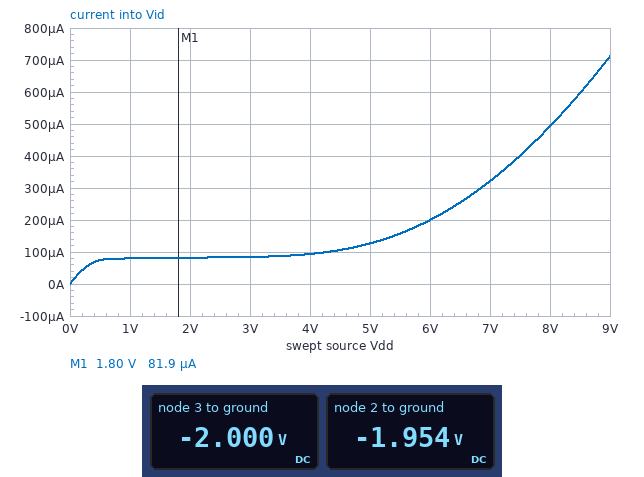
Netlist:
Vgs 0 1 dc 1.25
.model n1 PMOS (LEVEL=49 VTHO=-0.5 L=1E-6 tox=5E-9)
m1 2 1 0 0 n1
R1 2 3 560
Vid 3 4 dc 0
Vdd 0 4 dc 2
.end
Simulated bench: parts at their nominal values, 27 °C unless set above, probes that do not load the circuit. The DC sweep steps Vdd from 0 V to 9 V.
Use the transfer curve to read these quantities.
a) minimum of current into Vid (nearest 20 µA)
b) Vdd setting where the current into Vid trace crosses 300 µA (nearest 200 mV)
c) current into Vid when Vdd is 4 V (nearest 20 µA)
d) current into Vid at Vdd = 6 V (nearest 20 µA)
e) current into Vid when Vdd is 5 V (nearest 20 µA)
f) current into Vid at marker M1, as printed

0 A
6.8 V
100 µA
200 µA
120 µA
81.9 µA
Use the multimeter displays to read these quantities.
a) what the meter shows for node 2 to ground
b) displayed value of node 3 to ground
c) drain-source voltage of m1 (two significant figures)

-1.954 V
-2.000 V
-2.0 V
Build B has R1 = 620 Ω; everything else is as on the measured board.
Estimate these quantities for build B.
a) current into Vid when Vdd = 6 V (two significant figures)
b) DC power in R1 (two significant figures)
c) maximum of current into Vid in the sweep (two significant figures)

200 µA
4.2 µW
700 µA
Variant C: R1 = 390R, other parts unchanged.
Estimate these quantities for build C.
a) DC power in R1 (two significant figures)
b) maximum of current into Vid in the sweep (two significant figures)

2.6 µW
740 µA
